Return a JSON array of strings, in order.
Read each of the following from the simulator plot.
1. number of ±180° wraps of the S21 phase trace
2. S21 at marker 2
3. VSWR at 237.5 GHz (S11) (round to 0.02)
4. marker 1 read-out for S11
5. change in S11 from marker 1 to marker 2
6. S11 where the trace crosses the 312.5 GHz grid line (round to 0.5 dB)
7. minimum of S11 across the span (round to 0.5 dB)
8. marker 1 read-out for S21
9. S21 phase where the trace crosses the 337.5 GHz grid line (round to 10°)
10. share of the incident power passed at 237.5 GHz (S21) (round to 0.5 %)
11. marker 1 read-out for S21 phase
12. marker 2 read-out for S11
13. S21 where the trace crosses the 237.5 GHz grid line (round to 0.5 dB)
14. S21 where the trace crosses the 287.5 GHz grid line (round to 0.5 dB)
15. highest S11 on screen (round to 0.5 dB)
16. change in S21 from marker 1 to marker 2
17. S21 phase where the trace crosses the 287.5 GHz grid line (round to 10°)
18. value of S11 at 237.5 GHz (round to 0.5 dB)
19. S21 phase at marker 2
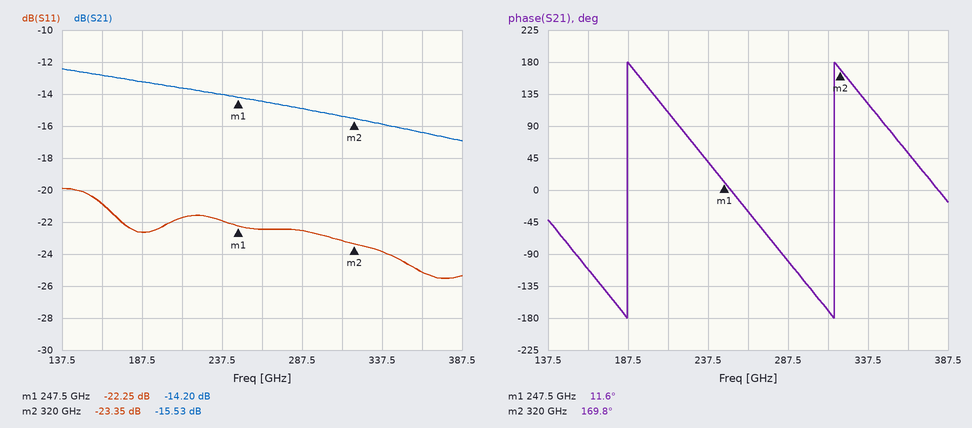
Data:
["2", "-15.53 dB", "1.18", "-22.25 dB", "-1.10 dB", "-23.0 dB", "-25.5 dB", "-14.20 dB", "120°", "4.0 %", "11.6°", "-23.35 dB", "-14.0 dB", "-15.0 dB", "-20.0 dB", "-1.33 dB", "-100°", "-22.0 dB", "169.8°"]
